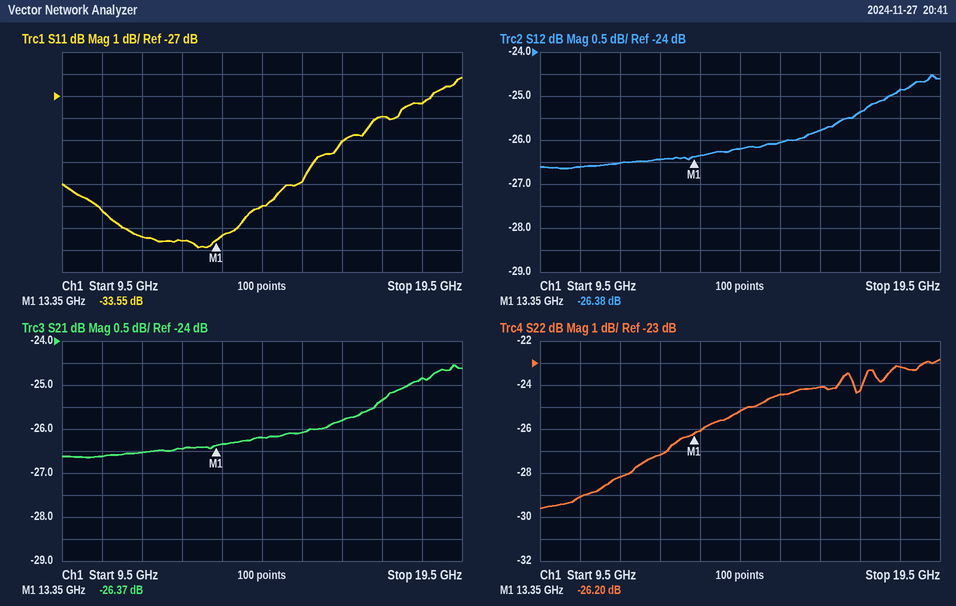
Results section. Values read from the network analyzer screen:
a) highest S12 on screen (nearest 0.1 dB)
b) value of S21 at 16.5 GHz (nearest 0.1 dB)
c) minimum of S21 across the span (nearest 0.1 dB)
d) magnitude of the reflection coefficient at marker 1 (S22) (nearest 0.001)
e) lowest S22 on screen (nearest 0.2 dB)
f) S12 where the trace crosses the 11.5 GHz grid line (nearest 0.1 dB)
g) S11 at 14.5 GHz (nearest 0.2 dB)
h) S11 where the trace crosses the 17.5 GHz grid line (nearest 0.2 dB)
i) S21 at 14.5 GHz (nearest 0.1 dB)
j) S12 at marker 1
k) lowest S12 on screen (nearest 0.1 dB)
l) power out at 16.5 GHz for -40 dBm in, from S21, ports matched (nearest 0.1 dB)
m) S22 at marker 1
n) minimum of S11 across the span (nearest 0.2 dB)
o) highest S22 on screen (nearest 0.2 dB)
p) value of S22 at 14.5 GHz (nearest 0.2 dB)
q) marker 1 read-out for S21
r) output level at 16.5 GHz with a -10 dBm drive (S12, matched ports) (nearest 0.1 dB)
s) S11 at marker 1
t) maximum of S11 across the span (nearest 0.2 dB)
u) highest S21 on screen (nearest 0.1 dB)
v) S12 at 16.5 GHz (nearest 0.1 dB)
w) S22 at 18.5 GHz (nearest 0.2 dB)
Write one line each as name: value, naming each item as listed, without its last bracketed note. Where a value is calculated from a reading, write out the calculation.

highest S12 on screen: -24.5 dB
value of S21 at 16.5 GHz: -25.8 dB
minimum of S21 across the span: -26.6 dB
magnitude of the reflection coefficient at marker 1 (S22): 10^(-26.2/20) ≈ 0.049
lowest S22 on screen: -29.6 dB
S12 where the trace crosses the 11.5 GHz grid line: -26.5 dB
S11 at 14.5 GHz: -32.0 dB
S11 where the trace crosses the 17.5 GHz grid line: -28.0 dB
S21 at 14.5 GHz: -26.2 dB
S12 at marker 1: -26.38 dB
lowest S12 on screen: -26.6 dB
power out at 16.5 GHz for -40 dBm in, from S21, ports matched: -40 dBm + (-25.8 dB) = -65.8 dBm
S22 at marker 1: -26.20 dB
minimum of S11 across the span: -33.8 dB
highest S22 on screen: -22.8 dB
value of S22 at 14.5 GHz: -25.2 dB
marker 1 read-out for S21: -26.37 dB
output level at 16.5 GHz with a -10 dBm drive (S12, matched ports): -10 dBm + (-25.8 dB) = -35.8 dBm
S11 at marker 1: -33.55 dB
maximum of S11 across the span: -26.2 dB
highest S21 on screen: -24.5 dB
S12 at 16.5 GHz: -25.8 dB
S22 at 18.5 GHz: -23.2 dB
